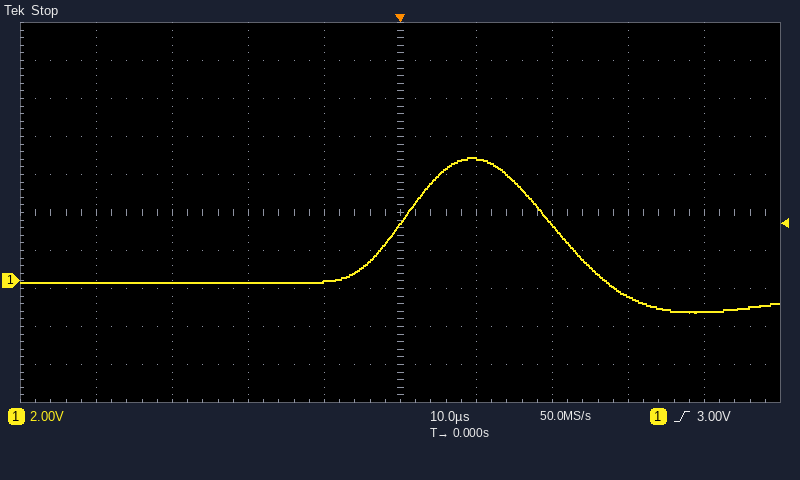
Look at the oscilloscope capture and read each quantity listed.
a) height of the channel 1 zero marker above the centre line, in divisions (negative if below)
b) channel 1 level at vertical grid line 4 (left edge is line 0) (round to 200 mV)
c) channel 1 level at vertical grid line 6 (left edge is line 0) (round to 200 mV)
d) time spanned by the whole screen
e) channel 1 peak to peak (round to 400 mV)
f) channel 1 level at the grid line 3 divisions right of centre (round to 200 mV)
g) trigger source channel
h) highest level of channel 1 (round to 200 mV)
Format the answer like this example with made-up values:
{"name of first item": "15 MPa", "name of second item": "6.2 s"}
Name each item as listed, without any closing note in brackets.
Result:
{"height of the channel 1 zero marker above the centre line, in divisions": "-1.8 div", "channel 1 level at vertical grid line 4 (left edge is line 0)": "0.0 V", "channel 1 level at vertical grid line 6 (left edge is line 0)": "6.4 V", "time spanned by the whole screen": "100 µs", "channel 1 peak to peak": "8.0 V", "channel 1 level at the grid line 3 divisions right of centre": "-800 mV", "trigger source channel": "channel 1", "highest level of channel 1": "6.4 V"}
